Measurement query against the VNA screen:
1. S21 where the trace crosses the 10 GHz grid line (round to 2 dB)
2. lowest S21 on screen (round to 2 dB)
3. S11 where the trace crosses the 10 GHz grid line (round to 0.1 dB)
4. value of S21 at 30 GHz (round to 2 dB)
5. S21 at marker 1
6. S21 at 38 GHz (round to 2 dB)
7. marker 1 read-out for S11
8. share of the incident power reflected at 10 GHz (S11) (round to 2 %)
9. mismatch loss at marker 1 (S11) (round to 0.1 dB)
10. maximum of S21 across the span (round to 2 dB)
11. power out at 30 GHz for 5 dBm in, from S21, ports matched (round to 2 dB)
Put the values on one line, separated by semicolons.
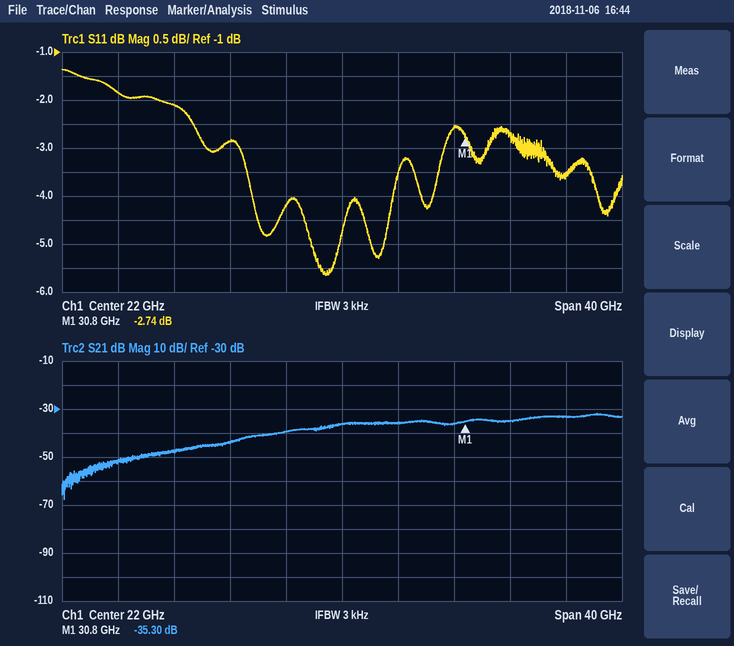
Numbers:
-48 dB; -68 dB; -2.1 dB; -36 dB; -35.30 dB; -34 dB; -2.74 dB; 62 %; 3.3 dB; -32 dB; -32 dBm
